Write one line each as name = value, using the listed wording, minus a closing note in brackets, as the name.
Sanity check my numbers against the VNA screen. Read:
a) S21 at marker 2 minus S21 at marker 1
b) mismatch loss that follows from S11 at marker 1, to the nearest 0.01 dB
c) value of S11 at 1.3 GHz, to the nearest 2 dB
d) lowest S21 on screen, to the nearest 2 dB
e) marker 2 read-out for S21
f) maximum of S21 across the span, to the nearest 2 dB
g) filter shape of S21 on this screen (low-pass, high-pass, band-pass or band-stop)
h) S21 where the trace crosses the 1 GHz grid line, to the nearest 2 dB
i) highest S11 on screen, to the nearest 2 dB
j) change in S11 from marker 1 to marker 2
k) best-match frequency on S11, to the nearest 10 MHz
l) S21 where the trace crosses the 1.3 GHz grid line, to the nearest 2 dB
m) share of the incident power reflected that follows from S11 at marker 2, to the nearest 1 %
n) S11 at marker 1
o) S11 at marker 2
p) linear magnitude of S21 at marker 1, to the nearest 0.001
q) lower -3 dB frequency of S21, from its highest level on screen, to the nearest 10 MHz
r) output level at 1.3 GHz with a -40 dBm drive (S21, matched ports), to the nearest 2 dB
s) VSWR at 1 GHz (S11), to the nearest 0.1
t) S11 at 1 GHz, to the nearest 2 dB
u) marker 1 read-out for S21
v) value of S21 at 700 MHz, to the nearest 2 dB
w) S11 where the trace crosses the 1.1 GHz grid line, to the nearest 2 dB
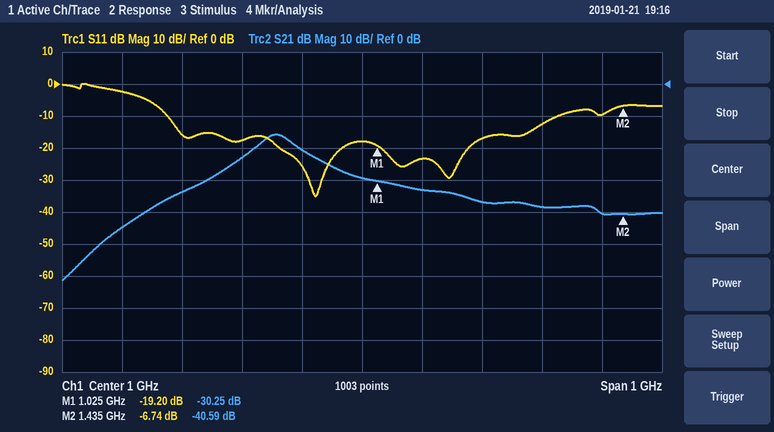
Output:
S21 at marker 2 minus S21 at marker 1 = -10.34 dB
mismatch loss that follows from S11 at marker 1, to the nearest 0.01 dB = 0.05 dB
value of S11 at 1.3 GHz, to the nearest 2 dB = -12 dB
lowest S21 on screen, to the nearest 2 dB = -62 dB
marker 2 read-out for S21 = -40.59 dB
maximum of S21 across the span, to the nearest 2 dB = -16 dB
filter shape of S21 on this screen = band-pass
S21 where the trace crosses the 1 GHz grid line, to the nearest 2 dB = -30 dB
highest S11 on screen, to the nearest 2 dB = 0 dB
change in S11 from marker 1 to marker 2 = 12.46 dB
best-match frequency on S11, to the nearest 10 MHz = 920 MHz
S21 where the trace crosses the 1.3 GHz grid line, to the nearest 2 dB = -38 dB
share of the incident power reflected that follows from S11 at marker 2, to the nearest 1 % = 21 %
S11 at marker 1 = -19.20 dB
S11 at marker 2 = -6.74 dB
linear magnitude of S21 at marker 1, to the nearest 0.001 = 0.031
lower -3 dB frequency of S21, from its highest level on screen, to the nearest 10 MHz = 830 MHz
output level at 1.3 GHz with a -40 dBm drive (S21, matched ports), to the nearest 2 dB = -78 dBm
VSWR at 1 GHz (S11), to the nearest 0.1 = 1.3
S11 at 1 GHz, to the nearest 2 dB = -18 dB
marker 1 read-out for S21 = -30.25 dB
value of S21 at 700 MHz, to the nearest 2 dB = -34 dB
S11 where the trace crosses the 1.1 GHz grid line, to the nearest 2 dB = -24 dB
